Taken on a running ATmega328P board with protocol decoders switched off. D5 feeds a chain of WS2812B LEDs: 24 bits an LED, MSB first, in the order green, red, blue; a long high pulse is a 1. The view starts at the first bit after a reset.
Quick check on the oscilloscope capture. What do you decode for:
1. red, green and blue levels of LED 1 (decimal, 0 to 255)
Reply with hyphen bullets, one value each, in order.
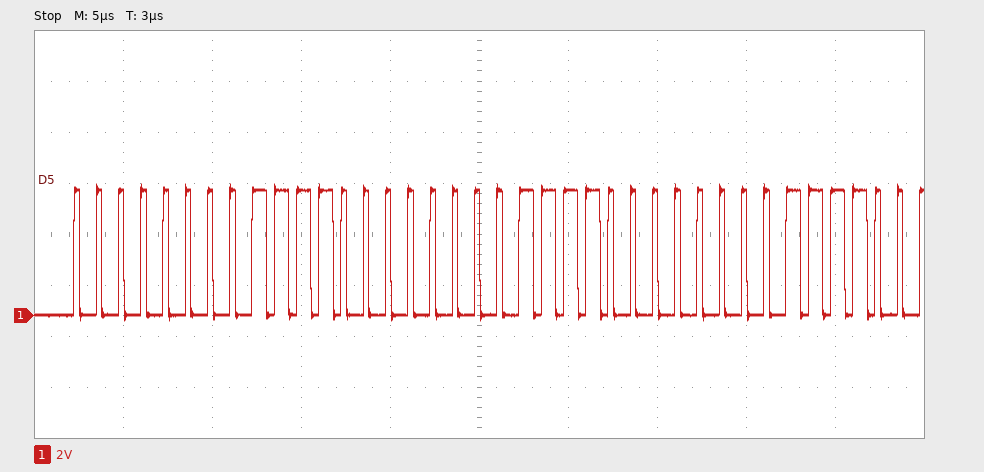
- 240, 0, 15
